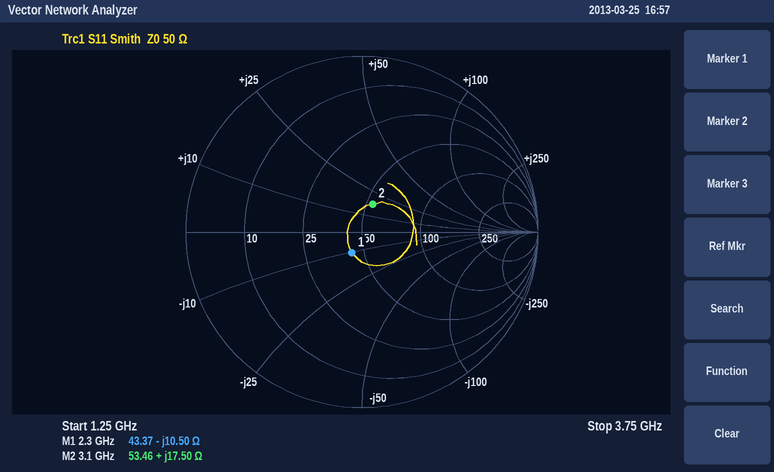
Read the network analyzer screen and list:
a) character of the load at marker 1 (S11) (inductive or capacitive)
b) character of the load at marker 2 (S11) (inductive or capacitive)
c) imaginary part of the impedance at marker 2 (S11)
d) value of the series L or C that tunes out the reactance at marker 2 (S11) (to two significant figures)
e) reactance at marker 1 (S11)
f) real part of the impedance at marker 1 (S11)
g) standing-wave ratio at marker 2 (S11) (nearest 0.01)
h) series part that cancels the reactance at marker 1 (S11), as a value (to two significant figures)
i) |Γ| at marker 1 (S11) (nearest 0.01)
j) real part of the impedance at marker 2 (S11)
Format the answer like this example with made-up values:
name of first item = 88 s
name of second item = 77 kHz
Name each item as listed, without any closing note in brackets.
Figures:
character of the load at marker 1 (S11) = capacitive
character of the load at marker 2 (S11) = inductive
imaginary part of the impedance at marker 2 = +17.50 Ω
value of the series L or C that tunes out the reactance at marker 2 (S11) = 2.9 pF
reactance at marker 1 = -10.50 Ω
real part of the impedance at marker 1 = 43.37 Ω
standing-wave ratio at marker 2 (S11) = 1.41
series part that cancels the reactance at marker 1 (S11), as a value = 730 pH
|Γ| at marker 1 (S11) = 0.13
real part of the impedance at marker 2 = 53.46 Ω
